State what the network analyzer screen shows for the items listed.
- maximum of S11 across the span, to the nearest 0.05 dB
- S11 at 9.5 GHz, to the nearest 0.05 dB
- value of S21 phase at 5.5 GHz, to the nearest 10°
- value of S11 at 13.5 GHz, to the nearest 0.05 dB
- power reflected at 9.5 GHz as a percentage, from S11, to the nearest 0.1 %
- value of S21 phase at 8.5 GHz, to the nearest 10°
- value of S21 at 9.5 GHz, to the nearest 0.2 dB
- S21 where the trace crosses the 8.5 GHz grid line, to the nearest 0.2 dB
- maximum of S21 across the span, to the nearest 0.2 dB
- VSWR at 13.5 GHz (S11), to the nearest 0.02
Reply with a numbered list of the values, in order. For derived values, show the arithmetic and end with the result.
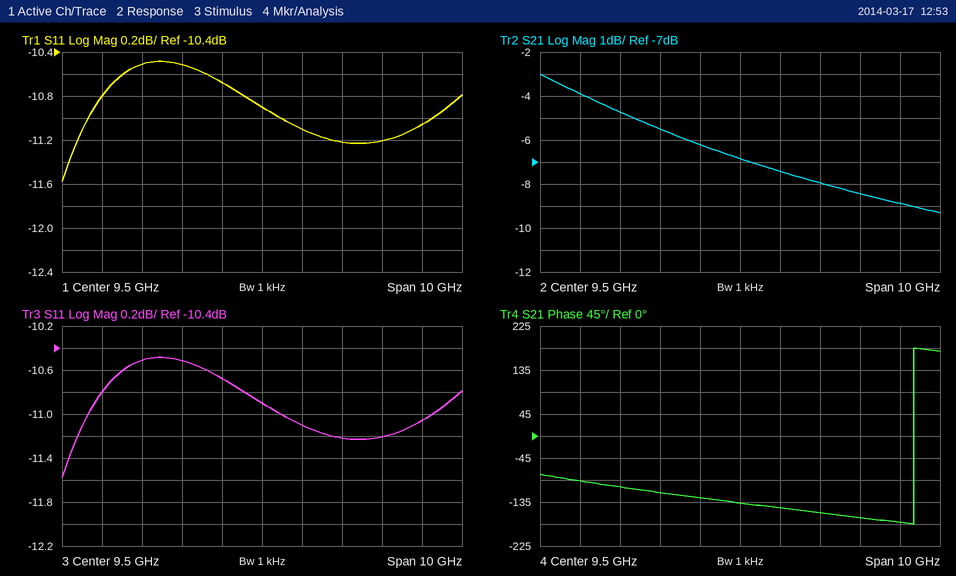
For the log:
1. -10.50 dB
2. -10.90 dB
3. -90°
4. -11.05 dB
5. 10^(-10.9/10) ≈ 8.1 %
6. -130°
7. -6.8 dB
8. -6.2 dB
9. -3.0 dB
10. |Γ| = 10^(-11.05/20) = 0.2802; VSWR = (1 + 0.2802)/(1 − 0.2802) ≈ 1.78
